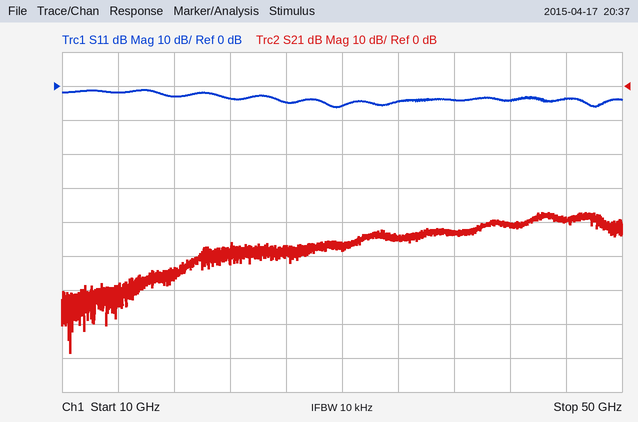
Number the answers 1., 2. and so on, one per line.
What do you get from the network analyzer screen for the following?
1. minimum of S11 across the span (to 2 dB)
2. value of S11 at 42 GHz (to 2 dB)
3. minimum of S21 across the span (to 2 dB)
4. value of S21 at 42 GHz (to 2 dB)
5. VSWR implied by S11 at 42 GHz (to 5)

1. -6 dB
2. -4 dB
3. -78 dB
4. -40 dB
5. 5
